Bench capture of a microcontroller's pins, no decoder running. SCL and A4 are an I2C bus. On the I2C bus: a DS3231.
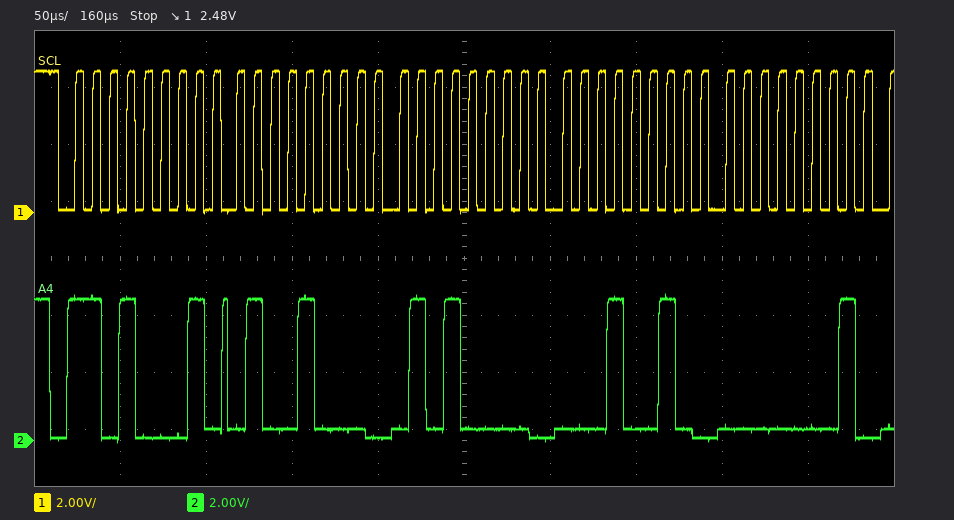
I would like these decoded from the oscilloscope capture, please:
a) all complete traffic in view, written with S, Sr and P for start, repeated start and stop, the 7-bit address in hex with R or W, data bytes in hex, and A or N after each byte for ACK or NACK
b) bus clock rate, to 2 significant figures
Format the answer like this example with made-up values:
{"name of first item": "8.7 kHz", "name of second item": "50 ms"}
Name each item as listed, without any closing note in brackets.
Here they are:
{"all complete traffic in view, written with S, Sr and P for start, repeated start and stop, the 7-bit address in hex with R or W, data bytes in hex, and A or N after each byte for ACK or NACK": "S 68R A 48 A 50 A 12 A 01 A", "bus clock rate, to 2 significant figures": "100 kHz"}
